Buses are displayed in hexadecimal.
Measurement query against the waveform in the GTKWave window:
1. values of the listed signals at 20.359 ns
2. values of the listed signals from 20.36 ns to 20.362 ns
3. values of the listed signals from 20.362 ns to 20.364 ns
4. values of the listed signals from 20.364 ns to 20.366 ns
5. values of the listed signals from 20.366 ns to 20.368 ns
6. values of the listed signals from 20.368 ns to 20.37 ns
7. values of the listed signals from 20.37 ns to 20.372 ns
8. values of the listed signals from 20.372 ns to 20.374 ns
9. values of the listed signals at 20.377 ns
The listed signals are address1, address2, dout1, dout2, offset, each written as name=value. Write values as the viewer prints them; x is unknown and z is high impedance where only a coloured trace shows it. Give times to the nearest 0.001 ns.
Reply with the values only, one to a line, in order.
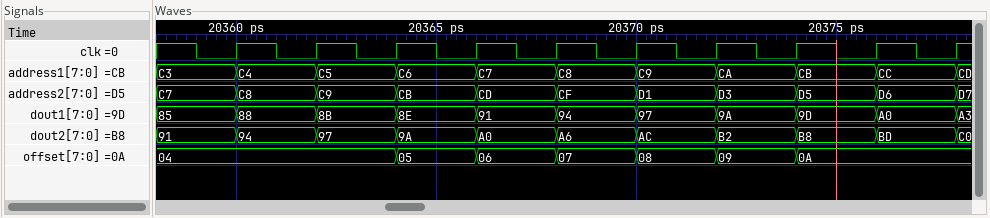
address1=C3, address2=C7, dout1=85, dout2=91, offset=04
address1=C4, address2=C8, dout1=88, dout2=94, offset=04
address1=C5, address2=C9, dout1=8B, dout2=97, offset=04
address1=C6, address2=CB, dout1=8E, dout2=9A, offset=05
address1=C7, address2=CD, dout1=91, dout2=A0, offset=06
address1=C8, address2=CF, dout1=94, dout2=A6, offset=07
address1=C9, address2=D1, dout1=97, dout2=AC, offset=08
address1=CA, address2=D3, dout1=9A, dout2=B2, offset=09
address1=CC, address2=D6, dout1=A0, dout2=BD, offset=0A
